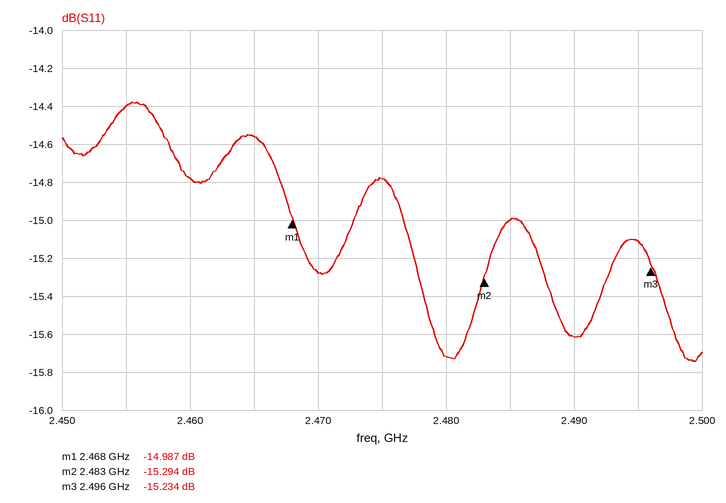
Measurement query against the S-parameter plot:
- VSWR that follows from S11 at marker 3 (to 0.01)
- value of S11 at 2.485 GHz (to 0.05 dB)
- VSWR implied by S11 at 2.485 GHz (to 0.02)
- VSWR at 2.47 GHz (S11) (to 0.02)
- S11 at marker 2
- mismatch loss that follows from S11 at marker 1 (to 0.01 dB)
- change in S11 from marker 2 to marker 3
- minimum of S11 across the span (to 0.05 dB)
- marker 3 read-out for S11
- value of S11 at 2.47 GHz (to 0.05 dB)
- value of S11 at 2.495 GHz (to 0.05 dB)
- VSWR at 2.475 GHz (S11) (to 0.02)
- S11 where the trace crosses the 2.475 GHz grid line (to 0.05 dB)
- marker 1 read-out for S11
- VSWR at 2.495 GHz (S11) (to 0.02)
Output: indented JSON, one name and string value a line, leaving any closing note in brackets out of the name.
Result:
{
  "VSWR that follows from S11 at marker 3": "1.42",
  "value of S11 at 2.485 GHz": "-15.00 dB",
  "VSWR implied by S11 at 2.485 GHz": "1.44",
  "VSWR at 2.47 GHz (S11)": "1.42",
  "S11 at marker 2": "-15.294 dB",
  "mismatch loss that follows from S11 at marker 1": "0.14 dB",
  "change in S11 from marker 2 to marker 3": "0.060 dB",
  "minimum of S11 across the span": "-15.75 dB",
  "marker 3 read-out for S11": "-15.234 dB",
  "value of S11 at 2.47 GHz": "-15.30 dB",
  "value of S11 at 2.495 GHz": "-15.10 dB",
  "VSWR at 2.475 GHz (S11)": "1.44",
  "S11 where the trace crosses the 2.475 GHz grid line": "-14.80 dB",
  "marker 1 read-out for S11": "-14.987 dB",
  "VSWR at 2.495 GHz (S11)": "1.42"
}
